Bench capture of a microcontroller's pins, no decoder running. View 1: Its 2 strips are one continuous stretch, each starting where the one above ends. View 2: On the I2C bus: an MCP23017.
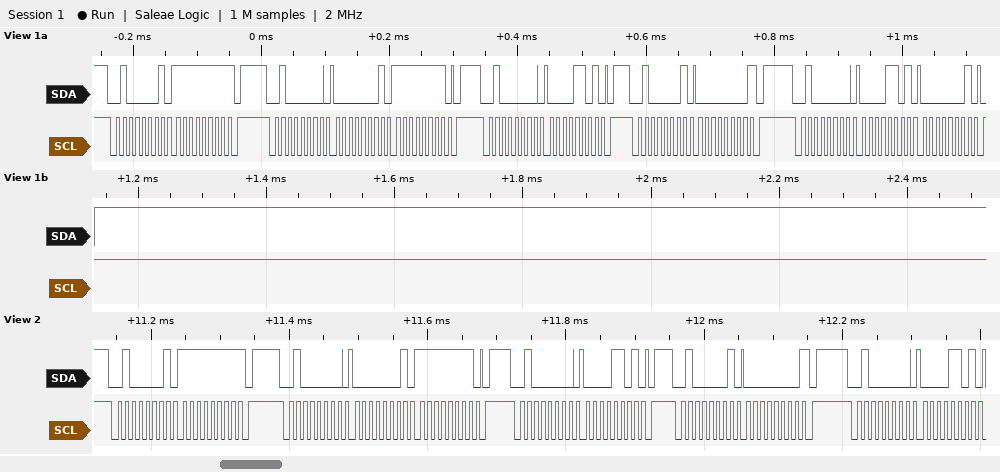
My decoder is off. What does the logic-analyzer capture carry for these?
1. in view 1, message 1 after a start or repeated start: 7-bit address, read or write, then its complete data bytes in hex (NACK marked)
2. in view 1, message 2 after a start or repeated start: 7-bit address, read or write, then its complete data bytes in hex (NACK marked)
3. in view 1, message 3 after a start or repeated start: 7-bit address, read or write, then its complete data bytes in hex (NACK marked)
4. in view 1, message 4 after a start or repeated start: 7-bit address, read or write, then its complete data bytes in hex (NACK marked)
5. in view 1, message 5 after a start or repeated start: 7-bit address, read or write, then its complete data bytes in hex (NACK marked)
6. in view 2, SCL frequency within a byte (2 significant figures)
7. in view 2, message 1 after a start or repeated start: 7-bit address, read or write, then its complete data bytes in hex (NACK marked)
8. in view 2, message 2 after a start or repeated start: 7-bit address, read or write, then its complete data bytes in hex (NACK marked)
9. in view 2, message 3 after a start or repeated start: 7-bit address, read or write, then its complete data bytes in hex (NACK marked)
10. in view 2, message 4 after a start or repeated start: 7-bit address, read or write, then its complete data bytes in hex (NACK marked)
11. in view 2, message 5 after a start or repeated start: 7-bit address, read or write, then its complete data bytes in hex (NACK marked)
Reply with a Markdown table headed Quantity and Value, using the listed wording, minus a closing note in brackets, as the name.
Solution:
| Quantity | Value |
|---|---|
| in view 1, message 1 after a start or repeated start: 7-bit address, read or write, then its complete data bytes in hex | 0x20 read: FF NACK |
| in view 1, message 2 after a start or repeated start: 7-bit address, read or write, then its complete data bytes in hex | 0x20 write: 01 FF |
| in view 1, message 3 after a start or repeated start: 7-bit address, read or write, then its complete data bytes in hex | 0x20 write: 0D |
| in view 1, message 4 after a start or repeated start: 7-bit address, read or write, then its complete data bytes in hex | 0x20 read: 00 NACK |
| in view 1, message 5 after a start or repeated start: 7-bit address, read or write, then its complete data bytes in hex | 0x20 write: 0D 01 |
| in view 2, SCL frequency within a byte | 100 kHz |
| in view 2, message 1 after a start or repeated start: 7-bit address, read or write, then its complete data bytes in hex | 0x20 read: FF NACK |
| in view 2, message 2 after a start or repeated start: 7-bit address, read or write, then its complete data bytes in hex | 0x20 write: 01 FF |
| in view 2, message 3 after a start or repeated start: 7-bit address, read or write, then its complete data bytes in hex | 0x20 write: 0D |
| in view 2, message 4 after a start or repeated start: 7-bit address, read or write, then its complete data bytes in hex | 0x20 read: 00 NACK |
| in view 2, message 5 after a start or repeated start: 7-bit address, read or write, then its complete data bytes in hex | 0x20 write: 0D |
